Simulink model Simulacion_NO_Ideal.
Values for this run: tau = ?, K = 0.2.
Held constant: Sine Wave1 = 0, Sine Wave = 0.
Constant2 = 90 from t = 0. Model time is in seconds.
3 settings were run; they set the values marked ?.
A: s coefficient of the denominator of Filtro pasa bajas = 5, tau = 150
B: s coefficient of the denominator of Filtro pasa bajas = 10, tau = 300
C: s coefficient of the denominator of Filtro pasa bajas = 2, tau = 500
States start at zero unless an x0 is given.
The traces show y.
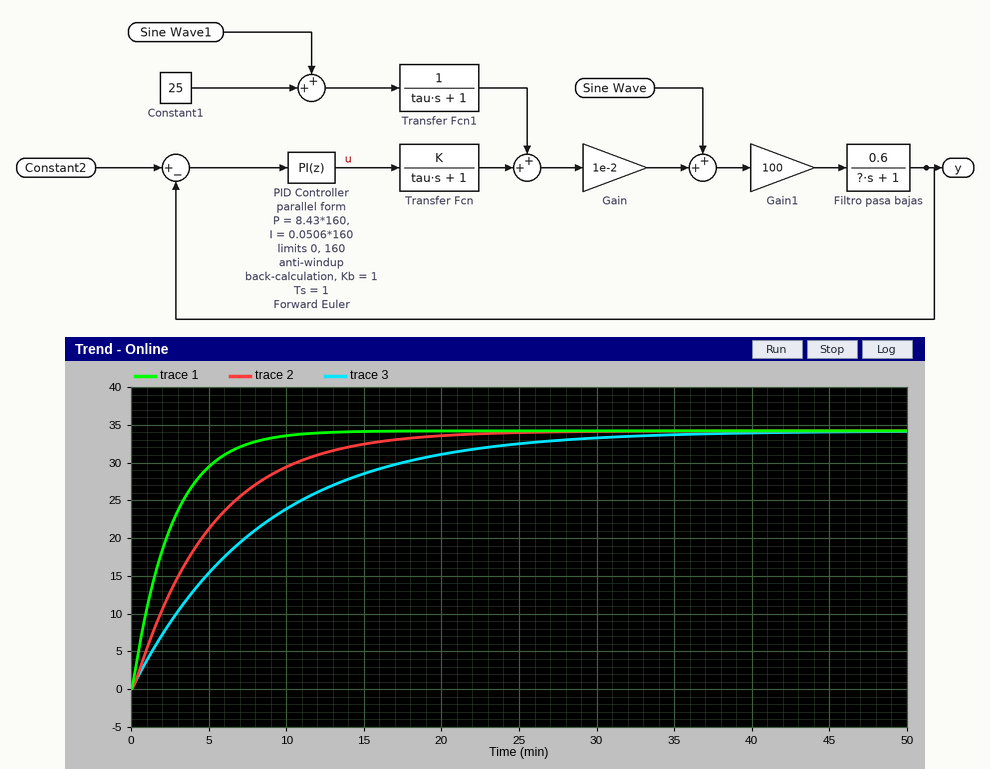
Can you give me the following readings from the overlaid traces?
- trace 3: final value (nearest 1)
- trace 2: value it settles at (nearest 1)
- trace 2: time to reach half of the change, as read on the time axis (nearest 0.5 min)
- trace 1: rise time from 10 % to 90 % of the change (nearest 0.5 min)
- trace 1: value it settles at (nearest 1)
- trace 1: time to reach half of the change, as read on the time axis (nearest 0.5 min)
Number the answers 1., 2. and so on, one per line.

1. 34
2. 34
3. 3.5 min
4. 5.5 min
5. 34
6. 2.0 min
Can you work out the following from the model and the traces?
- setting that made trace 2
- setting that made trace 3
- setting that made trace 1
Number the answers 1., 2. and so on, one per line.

1. B
2. C
3. A
